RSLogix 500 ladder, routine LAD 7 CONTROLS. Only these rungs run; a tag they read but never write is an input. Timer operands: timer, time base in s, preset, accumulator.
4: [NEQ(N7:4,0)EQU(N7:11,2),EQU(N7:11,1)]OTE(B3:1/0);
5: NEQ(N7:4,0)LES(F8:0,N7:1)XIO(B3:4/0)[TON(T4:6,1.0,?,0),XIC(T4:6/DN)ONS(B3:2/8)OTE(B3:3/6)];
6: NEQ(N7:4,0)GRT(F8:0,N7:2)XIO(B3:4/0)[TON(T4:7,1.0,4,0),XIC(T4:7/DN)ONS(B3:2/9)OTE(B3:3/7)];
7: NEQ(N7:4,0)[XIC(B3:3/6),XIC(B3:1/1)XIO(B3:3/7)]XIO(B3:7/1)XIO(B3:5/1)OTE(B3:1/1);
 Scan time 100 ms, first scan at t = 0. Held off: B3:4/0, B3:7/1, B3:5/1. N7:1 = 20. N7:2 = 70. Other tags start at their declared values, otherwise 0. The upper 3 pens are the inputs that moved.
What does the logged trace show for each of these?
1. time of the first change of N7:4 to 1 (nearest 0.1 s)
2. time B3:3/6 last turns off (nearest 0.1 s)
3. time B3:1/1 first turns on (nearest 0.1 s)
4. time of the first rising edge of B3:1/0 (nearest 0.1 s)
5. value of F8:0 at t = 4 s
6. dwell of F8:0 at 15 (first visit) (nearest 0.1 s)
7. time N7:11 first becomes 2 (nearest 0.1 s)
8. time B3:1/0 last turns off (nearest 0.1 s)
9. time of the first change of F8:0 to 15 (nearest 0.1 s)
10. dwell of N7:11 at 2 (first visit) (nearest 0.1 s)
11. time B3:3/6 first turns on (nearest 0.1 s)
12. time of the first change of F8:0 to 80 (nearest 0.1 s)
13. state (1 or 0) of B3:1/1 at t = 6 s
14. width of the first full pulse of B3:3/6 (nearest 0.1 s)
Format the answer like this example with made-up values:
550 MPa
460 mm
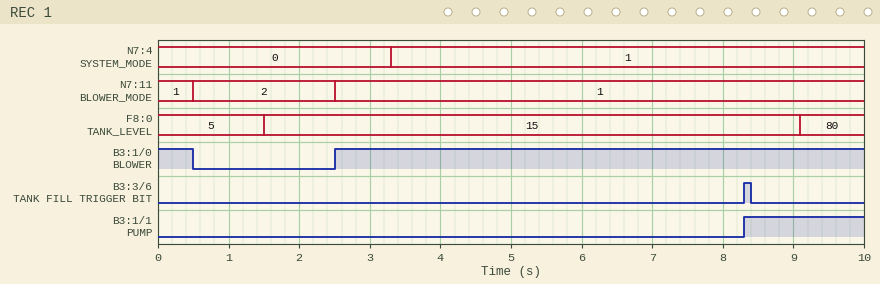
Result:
3.3 s
8.4 s
8.3 s
2.5 s
15
7.6 s
0.5 s
0.5 s
1.5 s
2.0 s
8.3 s
9.1 s
0
0.1 s
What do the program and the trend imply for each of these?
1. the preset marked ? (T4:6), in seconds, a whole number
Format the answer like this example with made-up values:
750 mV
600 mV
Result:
5 s
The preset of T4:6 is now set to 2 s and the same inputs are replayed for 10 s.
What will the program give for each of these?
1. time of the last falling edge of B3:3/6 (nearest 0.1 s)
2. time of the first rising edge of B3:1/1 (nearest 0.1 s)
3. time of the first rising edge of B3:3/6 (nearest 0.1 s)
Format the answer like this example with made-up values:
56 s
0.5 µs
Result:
5.4 s
5.3 s
5.3 s
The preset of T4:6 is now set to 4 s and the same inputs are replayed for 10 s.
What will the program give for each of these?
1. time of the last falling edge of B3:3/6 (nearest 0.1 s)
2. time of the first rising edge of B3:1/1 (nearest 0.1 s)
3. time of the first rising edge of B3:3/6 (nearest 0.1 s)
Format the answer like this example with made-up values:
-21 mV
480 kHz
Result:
7.4 s
7.3 s
7.3 s
